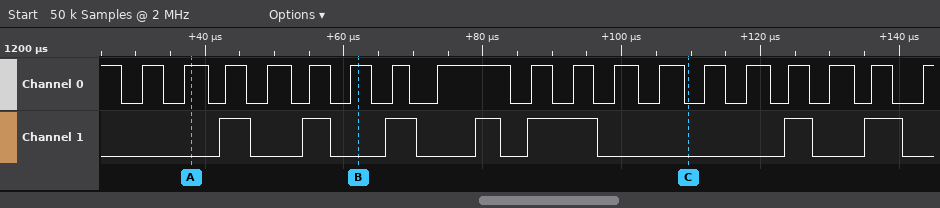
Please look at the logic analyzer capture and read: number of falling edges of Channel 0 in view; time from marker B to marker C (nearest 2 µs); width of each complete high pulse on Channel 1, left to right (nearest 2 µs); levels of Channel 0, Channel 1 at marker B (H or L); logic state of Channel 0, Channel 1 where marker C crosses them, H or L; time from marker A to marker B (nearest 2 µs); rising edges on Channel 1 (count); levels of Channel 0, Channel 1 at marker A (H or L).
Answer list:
18
48 µs
4 µs, 4 µs, 4 µs, 4 µs, 10 µs, 4 µs, 6 µs
Channel 0=H, Channel 1=L
Channel 0=L, Channel 1=L
24 µs
7
Channel 0=H, Channel 1=L
